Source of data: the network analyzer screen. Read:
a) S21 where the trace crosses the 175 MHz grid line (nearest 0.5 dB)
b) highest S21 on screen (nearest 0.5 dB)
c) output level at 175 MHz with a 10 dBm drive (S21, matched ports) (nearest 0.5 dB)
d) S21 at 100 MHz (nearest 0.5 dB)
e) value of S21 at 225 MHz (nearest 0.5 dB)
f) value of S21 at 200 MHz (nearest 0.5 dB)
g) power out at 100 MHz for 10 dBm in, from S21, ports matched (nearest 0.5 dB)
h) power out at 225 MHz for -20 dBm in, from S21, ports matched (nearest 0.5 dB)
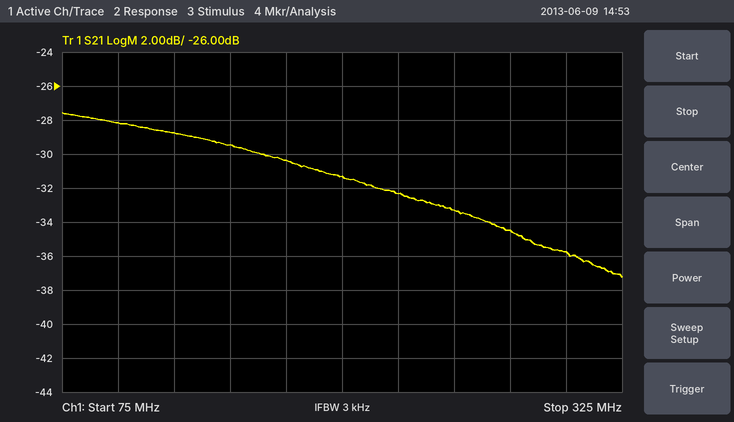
-30.5 dB
-27.5 dB
-20.5 dBm
-28.0 dB
-32.5 dB
-31.5 dB
-18.0 dBm
-52.5 dBm
